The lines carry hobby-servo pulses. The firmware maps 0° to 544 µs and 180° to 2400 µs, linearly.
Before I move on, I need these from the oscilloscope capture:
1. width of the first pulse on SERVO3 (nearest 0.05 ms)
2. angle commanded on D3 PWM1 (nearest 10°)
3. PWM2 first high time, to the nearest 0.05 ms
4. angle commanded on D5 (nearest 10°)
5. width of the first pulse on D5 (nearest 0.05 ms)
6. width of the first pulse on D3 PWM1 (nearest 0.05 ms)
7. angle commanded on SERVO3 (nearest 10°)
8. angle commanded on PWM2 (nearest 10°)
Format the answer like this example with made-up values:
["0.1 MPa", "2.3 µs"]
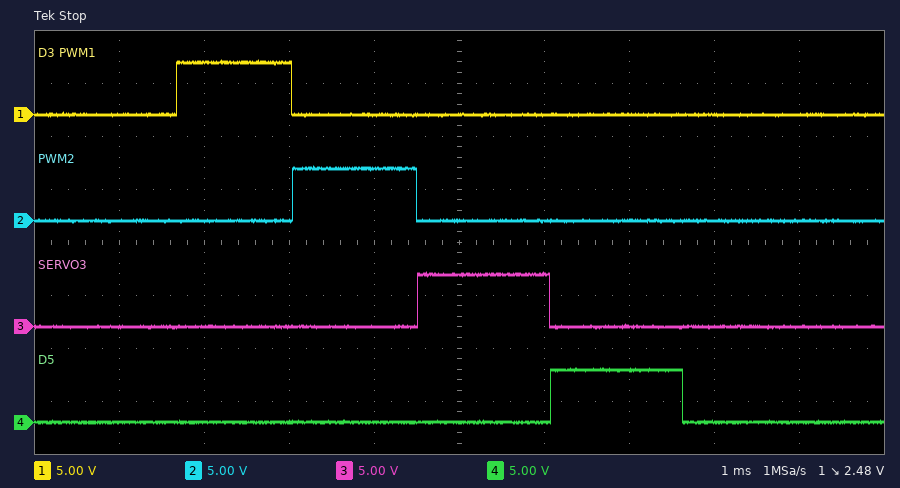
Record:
["1.55 ms", "80°", "1.45 ms", "100°", "1.55 ms", "1.35 ms", "100°", "90°"]
